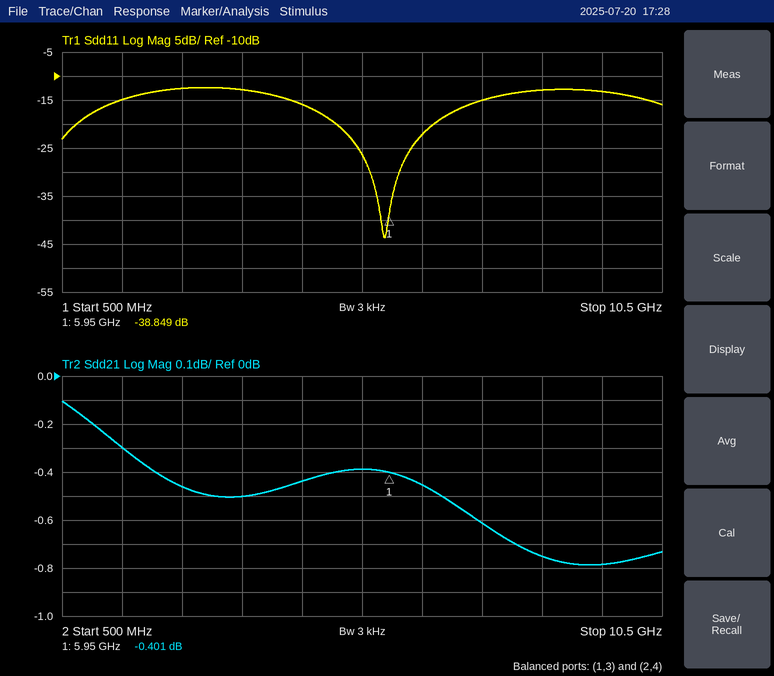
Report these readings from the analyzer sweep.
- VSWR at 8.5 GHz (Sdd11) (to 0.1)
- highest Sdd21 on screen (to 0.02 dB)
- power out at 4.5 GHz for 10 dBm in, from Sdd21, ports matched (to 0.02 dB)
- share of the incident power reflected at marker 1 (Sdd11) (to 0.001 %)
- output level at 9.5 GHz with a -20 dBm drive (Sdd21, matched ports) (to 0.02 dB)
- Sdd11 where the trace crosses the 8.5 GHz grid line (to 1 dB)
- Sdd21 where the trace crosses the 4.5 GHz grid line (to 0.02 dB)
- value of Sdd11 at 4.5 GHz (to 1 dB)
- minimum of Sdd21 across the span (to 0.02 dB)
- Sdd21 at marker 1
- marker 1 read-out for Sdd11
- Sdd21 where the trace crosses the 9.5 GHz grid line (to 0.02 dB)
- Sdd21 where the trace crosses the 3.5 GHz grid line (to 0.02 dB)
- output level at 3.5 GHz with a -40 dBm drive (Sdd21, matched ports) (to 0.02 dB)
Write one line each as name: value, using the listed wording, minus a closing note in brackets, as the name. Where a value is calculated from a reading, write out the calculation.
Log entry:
VSWR at 8.5 GHz (Sdd11): |Γ| = 10^(-13/20) = 0.2239; VSWR = (1 + 0.2239)/(1 − 0.2239) ≈ 1.6
highest Sdd21 on screen: -0.10 dB
power out at 4.5 GHz for 10 dBm in, from Sdd21, ports matched: 10 dBm + (-0.44 dB) = 9.56 dBm
share of the incident power reflected at marker 1 (Sdd11): 10^(-38.849/10) ≈ 0.013 %
output level at 9.5 GHz with a -20 dBm drive (Sdd21, matched ports): -20 dBm + (-0.78 dB) = -20.78 dBm
Sdd11 where the trace crosses the 8.5 GHz grid line: -13 dB
Sdd21 where the trace crosses the 4.5 GHz grid line: -0.44 dB
value of Sdd11 at 4.5 GHz: -16 dB
minimum of Sdd21 across the span: -0.78 dB
Sdd21 at marker 1: -0.401 dB
marker 1 read-out for Sdd11: -38.849 dB
Sdd21 where the trace crosses the 9.5 GHz grid line: -0.78 dB
Sdd21 where the trace crosses the 3.5 GHz grid line: -0.50 dB
output level at 3.5 GHz with a -40 dBm drive (Sdd21, matched ports): -40 dBm + (-0.50 dB) = -40.50 dBm
